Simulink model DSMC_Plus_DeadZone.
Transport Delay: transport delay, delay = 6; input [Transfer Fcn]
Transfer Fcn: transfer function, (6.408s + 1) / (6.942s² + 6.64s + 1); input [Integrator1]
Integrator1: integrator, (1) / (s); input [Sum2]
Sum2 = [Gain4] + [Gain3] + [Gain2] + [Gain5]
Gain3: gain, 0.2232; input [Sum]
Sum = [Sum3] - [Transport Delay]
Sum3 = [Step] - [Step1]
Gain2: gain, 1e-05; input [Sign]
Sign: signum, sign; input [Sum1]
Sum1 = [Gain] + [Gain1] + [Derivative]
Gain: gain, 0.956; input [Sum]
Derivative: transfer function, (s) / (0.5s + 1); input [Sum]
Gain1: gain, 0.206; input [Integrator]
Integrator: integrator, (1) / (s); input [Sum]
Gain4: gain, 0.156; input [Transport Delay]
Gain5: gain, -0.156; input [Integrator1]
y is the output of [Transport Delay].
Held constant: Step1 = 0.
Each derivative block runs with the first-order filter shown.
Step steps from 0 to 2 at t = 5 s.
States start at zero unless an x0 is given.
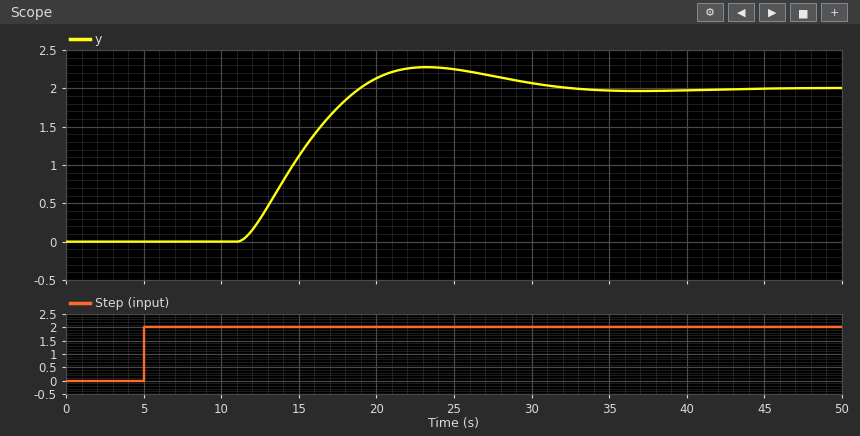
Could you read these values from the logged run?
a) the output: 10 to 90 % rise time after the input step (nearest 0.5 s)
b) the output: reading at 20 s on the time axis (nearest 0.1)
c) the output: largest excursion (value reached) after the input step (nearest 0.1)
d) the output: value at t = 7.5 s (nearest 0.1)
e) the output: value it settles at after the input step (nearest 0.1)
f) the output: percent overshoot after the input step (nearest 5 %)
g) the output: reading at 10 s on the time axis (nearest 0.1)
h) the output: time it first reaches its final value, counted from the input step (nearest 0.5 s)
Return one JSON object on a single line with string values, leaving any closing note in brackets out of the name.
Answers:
{"the output: 10 to 90 % rise time after the input step": "5.5 s", "the output: reading at 20 s on the time axis": "2.1", "the output: largest excursion (value reached) after the input step": "2.3", "the output: value at t = 7.5 s": "0.0", "the output: value it settles at after the input step": "2.0", "the output: percent overshoot after the input step": "15 %", "the output: reading at 10 s on the time axis": "0.0", "the output: time it first reaches its final value, counted from the input step": "14.0 s"}
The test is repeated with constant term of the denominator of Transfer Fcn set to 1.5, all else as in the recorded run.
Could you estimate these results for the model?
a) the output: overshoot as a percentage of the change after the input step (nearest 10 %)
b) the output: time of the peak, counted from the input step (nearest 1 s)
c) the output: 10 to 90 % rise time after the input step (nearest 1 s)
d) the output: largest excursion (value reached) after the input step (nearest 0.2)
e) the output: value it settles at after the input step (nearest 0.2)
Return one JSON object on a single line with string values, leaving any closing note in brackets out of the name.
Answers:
{"the output: overshoot as a percentage of the change after the input step": "20 %", "the output: time of the peak, counted from the input step": "16 s", "the output: 10 to 90 % rise time after the input step": "4 s", "the output: largest excursion (value reached) after the input step": "1.8", "the output: value it settles at after the input step": "1.4"}
